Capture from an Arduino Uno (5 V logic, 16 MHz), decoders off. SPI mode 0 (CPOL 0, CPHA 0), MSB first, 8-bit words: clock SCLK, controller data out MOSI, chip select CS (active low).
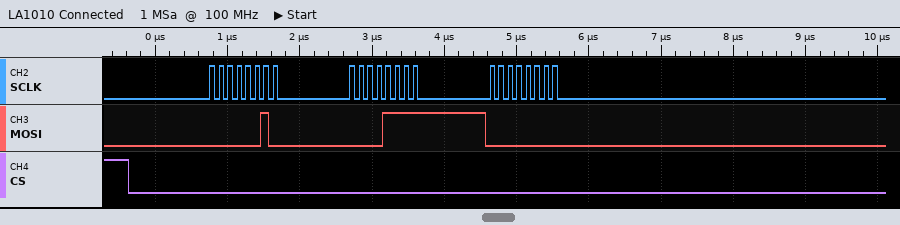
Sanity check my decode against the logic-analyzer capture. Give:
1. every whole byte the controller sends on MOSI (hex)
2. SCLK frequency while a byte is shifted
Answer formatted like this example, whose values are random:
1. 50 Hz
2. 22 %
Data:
1. 02 0F 00
2. 8 MHz
